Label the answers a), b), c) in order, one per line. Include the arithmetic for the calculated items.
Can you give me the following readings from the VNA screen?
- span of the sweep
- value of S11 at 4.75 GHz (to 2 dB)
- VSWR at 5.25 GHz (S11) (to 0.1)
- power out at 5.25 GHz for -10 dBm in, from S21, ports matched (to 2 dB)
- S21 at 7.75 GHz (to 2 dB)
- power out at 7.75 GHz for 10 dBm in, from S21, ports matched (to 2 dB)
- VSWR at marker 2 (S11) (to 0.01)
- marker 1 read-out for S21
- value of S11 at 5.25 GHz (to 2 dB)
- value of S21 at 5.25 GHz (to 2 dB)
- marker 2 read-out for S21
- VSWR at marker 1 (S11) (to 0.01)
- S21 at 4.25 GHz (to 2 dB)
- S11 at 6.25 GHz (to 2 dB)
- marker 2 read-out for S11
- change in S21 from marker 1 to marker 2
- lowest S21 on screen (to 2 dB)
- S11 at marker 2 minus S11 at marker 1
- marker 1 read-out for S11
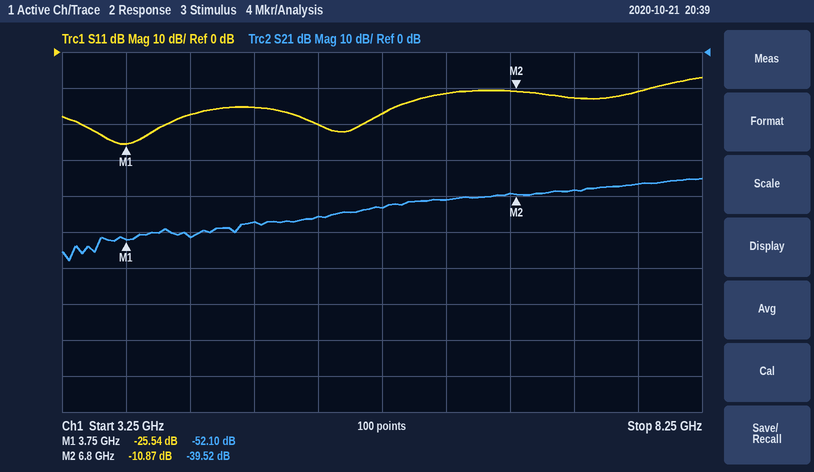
a) 5 GHz
b) -16 dB
c) |Γ| = 10^(-20/20) = 0.1000; VSWR = (1 + 0.1000)/(1 − 0.1000) ≈ 1.2
d) -10 dBm + (-46 dB) = -56 dBm
e) -36 dB
f) 10 dBm + (-36 dB) = -26 dBm
g) (1 + 0.2861)/(1 − 0.2861) ≈ 1.80
h) -52.10 dB
i) -20 dB
j) -46 dB
k) -39.52 dB
l) (1 + 0.0528)/(1 − 0.0528) ≈ 1.11
m) -52 dB
n) -12 dB
o) -10.87 dB
p) -39.52 − (-52.1) = 12.58 dB
q) -58 dB
r) -10.87 − (-25.54) = 14.67 dB
s) -25.54 dB
